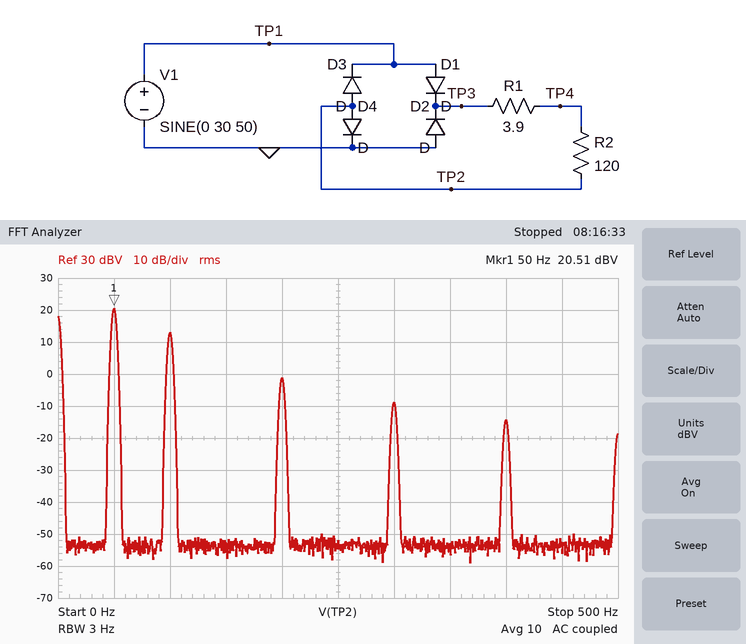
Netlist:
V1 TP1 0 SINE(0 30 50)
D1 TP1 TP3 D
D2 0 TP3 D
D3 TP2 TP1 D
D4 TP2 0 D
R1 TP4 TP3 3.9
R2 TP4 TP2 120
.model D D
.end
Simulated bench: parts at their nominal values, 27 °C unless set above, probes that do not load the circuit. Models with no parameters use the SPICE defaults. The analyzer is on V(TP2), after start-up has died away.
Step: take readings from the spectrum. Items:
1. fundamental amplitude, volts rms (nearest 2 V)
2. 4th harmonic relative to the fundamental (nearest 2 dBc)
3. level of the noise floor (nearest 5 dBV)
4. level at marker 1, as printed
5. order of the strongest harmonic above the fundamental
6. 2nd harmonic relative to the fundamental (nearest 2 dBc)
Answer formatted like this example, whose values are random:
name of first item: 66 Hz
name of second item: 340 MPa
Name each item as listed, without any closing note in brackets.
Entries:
fundamental amplitude, volts rms: 10 V
4th harmonic relative to the fundamental: -22 dBc
level of the noise floor: -55 dBV
level at marker 1, as printed: 20.51 dBV
order of the strongest harmonic above the fundamental: 2
2nd harmonic relative to the fundamental: -8 dBc
